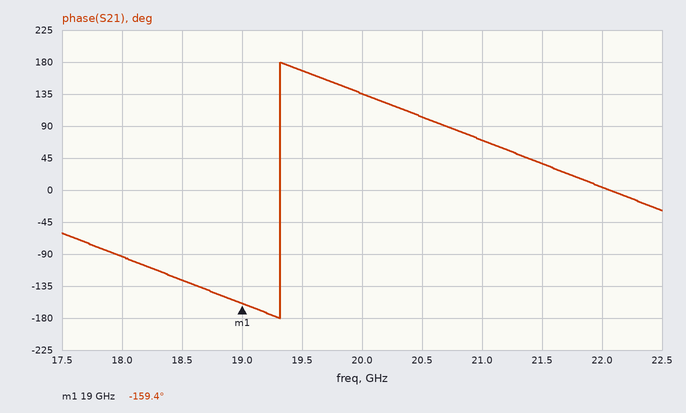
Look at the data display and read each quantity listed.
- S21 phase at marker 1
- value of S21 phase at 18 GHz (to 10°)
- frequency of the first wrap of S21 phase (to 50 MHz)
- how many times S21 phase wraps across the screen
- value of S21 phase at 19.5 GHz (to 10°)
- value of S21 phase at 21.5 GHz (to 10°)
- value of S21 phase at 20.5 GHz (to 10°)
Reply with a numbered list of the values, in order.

1. -159.4°
2. -90°
3. 19.30 GHz
4. 1
5. 170°
6. 40°
7. 100°
